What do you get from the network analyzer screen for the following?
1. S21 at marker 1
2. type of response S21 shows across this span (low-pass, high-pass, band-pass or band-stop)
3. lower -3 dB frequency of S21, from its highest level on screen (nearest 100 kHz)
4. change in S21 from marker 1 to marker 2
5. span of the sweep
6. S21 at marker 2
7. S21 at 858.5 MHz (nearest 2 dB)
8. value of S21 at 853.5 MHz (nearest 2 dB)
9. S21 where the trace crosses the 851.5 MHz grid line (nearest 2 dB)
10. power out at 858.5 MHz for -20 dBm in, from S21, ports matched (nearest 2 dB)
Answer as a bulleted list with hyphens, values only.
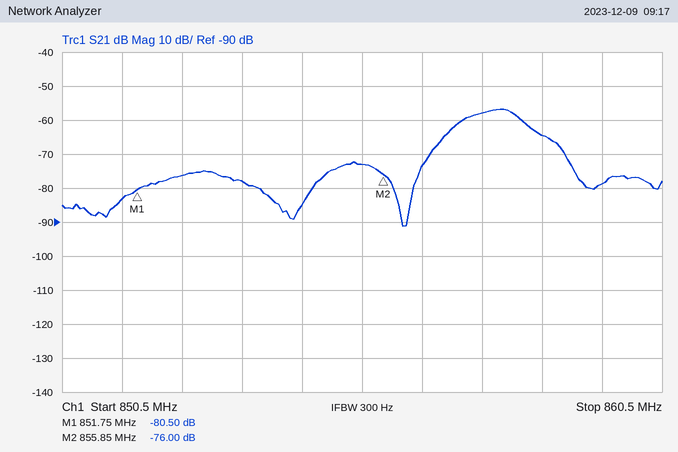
- -80.50 dB
- band-pass
- 857.2 MHz
- 4.50 dB
- 10 MHz
- -76.00 dB
- -64 dB
- -78 dB
- -84 dB
- -84 dBm
